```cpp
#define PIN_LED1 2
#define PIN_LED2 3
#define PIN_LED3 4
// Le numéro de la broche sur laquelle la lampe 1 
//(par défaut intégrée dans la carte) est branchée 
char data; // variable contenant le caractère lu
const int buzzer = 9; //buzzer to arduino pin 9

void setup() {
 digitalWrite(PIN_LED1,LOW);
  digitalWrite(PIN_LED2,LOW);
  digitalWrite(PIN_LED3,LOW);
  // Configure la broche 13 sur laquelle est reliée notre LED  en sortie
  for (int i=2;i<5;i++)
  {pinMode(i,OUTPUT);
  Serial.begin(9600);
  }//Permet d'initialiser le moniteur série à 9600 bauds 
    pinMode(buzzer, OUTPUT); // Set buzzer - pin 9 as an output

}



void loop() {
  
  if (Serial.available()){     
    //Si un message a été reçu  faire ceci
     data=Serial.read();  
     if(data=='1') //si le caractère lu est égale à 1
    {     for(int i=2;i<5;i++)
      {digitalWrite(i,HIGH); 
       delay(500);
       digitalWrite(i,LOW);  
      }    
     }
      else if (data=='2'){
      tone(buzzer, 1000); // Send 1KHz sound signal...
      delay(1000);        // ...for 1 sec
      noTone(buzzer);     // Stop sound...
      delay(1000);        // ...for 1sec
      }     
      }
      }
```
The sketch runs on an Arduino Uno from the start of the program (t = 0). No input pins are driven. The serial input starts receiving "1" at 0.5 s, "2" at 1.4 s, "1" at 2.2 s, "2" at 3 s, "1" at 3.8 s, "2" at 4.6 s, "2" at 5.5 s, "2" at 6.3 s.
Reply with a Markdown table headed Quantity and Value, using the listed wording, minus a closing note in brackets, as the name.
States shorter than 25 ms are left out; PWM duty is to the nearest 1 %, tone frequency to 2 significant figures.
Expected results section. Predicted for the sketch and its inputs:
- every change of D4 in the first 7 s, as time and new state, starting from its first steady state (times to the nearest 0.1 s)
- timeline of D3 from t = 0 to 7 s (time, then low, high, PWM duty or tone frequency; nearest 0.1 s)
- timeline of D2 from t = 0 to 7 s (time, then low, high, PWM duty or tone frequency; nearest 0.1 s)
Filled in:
| Quantity | Value |
|---|---|
| every change of D4 in the first 7 s, as time and new state, starting from its first steady state | 0 s low; 1.5 s high; 2 s low; 5 s high; 5.5 s low |
| timeline of D3 from t = 0 to 7 s | 0 s low; 1 s high; 1.5 s low; 4.5 s high; 5 s low |
| timeline of D2 from t = 0 to 7 s | 0 s low; 0.5 s high; 1 s low; 4 s high; 4.5 s low |
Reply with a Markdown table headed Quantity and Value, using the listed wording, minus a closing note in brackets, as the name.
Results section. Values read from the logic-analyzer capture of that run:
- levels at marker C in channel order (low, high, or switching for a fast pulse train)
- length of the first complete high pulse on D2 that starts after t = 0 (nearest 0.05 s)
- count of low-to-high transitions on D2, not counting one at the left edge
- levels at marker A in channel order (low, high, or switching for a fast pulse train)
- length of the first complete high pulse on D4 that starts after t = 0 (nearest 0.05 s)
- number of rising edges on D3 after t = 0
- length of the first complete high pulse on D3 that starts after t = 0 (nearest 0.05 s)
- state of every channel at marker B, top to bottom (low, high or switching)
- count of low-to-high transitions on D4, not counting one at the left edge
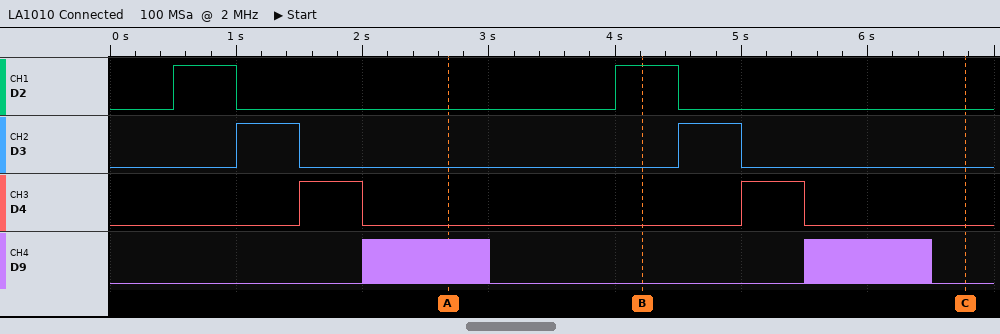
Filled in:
| Quantity | Value |
|---|---|
| levels at marker C in channel order | D2 low, D3 low, D4 low, D9 low |
| length of the first complete high pulse on D2 that starts after t = 0 | 0.50 s |
| count of low-to-high transitions on D2, not counting one at the left edge | 2 |
| levels at marker A in channel order | D2 low, D3 low, D4 low, D9 switching |
| length of the first complete high pulse on D4 that starts after t = 0 | 0.50 s |
| number of rising edges on D3 after t = 0 | 2 |
| length of the first complete high pulse on D3 that starts after t = 0 | 0.50 s |
| state of every channel at marker B, top to bottom | D2 high, D3 low, D4 low, D9 low |
| count of low-to-high transitions on D4, not counting one at the left edge | 2 |
